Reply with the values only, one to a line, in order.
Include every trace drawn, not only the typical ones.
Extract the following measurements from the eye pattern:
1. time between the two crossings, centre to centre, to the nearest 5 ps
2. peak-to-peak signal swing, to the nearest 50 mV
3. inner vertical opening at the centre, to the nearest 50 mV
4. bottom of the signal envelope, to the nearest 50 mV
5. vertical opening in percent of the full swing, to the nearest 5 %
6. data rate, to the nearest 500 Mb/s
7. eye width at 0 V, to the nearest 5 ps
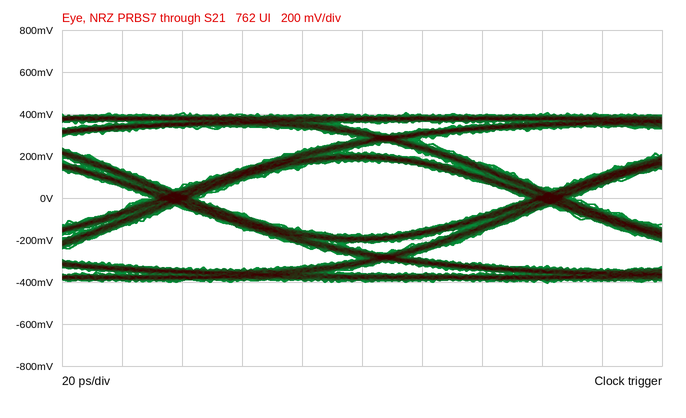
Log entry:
125 ps
800 mV
350 mV
-400 mV
45 %
8.0 Gb/s
110 ps
